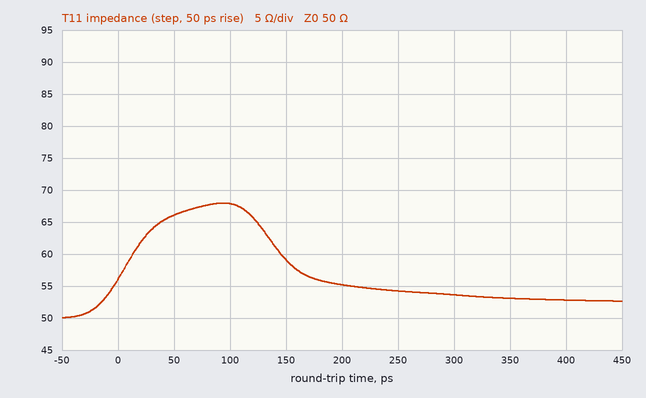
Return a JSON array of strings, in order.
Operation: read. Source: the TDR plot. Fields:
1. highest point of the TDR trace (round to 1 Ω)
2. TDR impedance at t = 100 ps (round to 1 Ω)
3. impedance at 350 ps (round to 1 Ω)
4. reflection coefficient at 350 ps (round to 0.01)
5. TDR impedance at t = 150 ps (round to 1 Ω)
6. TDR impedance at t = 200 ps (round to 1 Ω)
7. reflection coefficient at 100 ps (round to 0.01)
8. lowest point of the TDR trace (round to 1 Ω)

["68 Ω", "68 Ω", "53 Ω", "+0.03", "59 Ω", "55 Ω", "+0.15", "50 Ω"]
